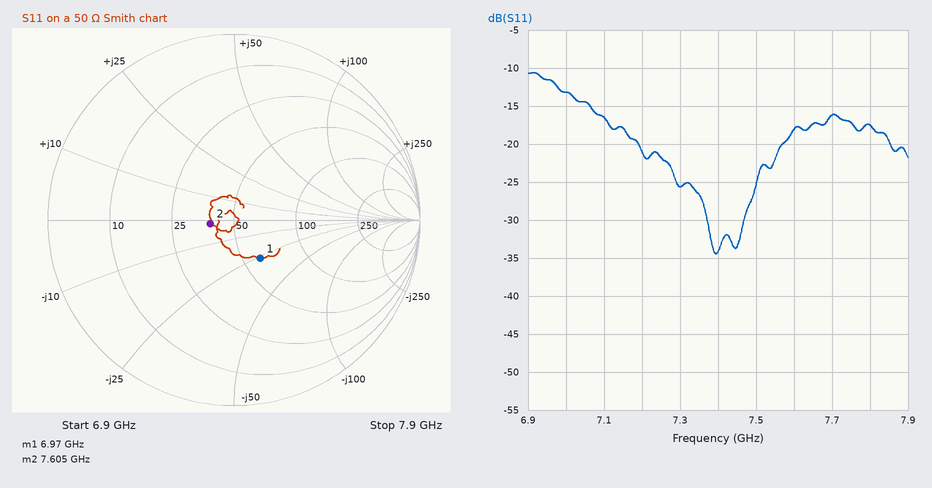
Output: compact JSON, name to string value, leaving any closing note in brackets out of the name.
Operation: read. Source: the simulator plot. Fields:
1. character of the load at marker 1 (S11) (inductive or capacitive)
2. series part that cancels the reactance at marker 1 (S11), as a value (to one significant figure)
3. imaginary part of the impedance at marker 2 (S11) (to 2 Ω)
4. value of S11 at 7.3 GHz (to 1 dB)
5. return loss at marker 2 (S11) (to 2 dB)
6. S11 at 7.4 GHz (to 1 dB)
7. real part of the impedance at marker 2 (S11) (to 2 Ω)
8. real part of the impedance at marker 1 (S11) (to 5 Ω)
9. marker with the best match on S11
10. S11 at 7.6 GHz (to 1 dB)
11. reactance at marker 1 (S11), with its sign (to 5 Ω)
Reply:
{"character of the load at marker 1 (S11)": "capacitive", "series part that cancels the reactance at marker 1 (S11), as a value": "600 pH", "imaginary part of the impedance at marker 2 (S11)": "-2 Ω", "value of S11 at 7.3 GHz": "-26 dB", "return loss at marker 2 (S11)": "18 dB", "S11 at 7.4 GHz": "-34 dB", "real part of the impedance at marker 2 (S11)": "38 Ω", "real part of the impedance at marker 1 (S11)": "60 Ω", "marker with the best match on S11": "marker 2", "S11 at 7.6 GHz": "-18 dB", "reactance at marker 1 (S11), with its sign": "-25 Ω"}
